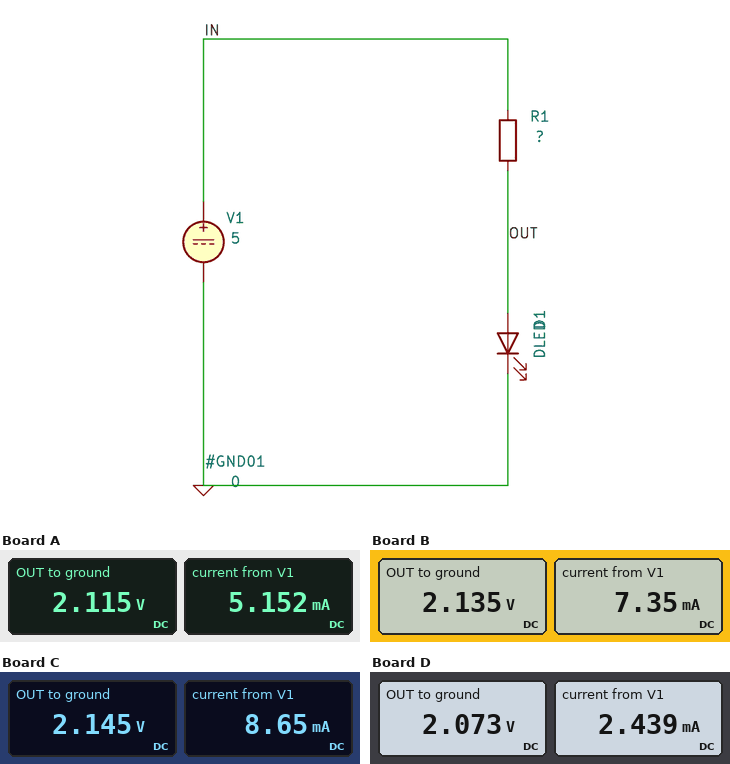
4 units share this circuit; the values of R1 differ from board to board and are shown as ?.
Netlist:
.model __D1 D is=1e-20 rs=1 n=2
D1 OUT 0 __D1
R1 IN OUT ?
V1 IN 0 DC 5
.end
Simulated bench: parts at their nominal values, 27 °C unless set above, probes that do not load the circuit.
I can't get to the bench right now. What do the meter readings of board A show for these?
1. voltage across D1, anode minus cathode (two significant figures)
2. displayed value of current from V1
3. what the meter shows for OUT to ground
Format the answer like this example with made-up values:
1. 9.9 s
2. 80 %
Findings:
1. 2.1 V
2. 5.152 mA
3. 2.115 V
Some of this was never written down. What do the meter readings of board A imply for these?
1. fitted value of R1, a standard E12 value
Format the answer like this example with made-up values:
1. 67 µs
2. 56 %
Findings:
1. 560 Ω
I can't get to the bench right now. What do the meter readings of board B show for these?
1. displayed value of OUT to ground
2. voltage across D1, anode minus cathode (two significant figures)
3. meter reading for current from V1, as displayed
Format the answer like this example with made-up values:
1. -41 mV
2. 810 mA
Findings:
1. 2.135 V
2. 2.1 V
3. 7.35 mA
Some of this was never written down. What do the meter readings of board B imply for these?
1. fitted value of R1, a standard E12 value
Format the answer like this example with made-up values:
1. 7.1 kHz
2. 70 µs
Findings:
1. 390 Ω
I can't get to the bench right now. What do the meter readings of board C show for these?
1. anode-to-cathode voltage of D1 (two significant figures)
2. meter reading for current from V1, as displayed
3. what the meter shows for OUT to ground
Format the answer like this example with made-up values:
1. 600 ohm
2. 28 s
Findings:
1. 2.1 V
2. 8.65 mA
3. 2.145 V
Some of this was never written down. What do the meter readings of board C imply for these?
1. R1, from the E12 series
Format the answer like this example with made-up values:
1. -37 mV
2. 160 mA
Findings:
1. 330 Ω
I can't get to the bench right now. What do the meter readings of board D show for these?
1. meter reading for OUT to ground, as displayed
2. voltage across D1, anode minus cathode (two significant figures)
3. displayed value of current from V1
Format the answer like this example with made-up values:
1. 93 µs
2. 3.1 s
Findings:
1. 2.073 V
2. 2.1 V
3. 2.439 mA
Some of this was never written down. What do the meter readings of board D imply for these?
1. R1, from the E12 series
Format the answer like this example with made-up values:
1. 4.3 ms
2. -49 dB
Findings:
1. 1.2 kΩ
